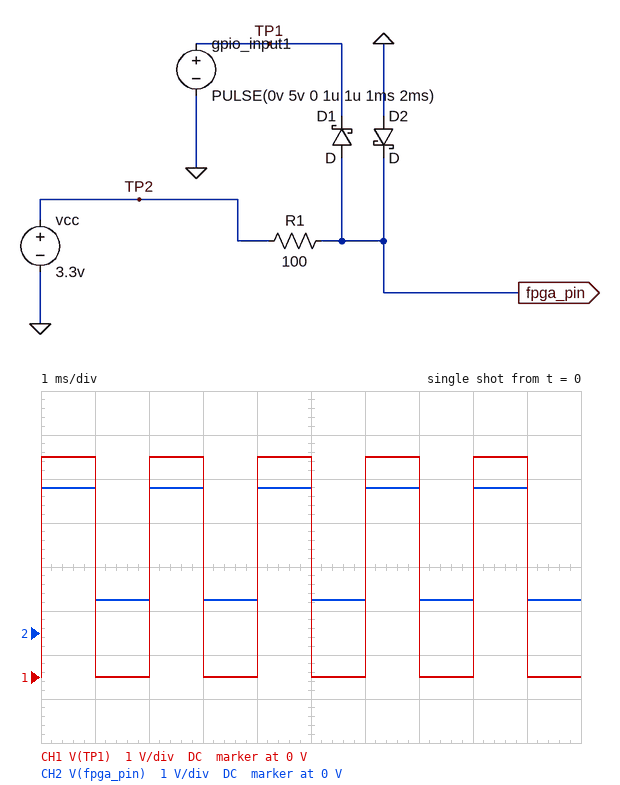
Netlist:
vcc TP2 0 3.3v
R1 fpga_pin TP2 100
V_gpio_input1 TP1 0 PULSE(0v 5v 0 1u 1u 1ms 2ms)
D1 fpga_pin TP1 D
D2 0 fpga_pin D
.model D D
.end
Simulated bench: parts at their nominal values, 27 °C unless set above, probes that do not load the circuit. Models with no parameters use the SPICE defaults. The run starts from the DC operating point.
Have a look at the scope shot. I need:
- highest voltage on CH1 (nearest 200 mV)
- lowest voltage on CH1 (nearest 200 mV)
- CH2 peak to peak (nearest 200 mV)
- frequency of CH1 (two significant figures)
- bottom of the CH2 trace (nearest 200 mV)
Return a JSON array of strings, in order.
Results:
["5.0 V", "0 V", "2.6 V", "500 Hz", "800 mV"]
